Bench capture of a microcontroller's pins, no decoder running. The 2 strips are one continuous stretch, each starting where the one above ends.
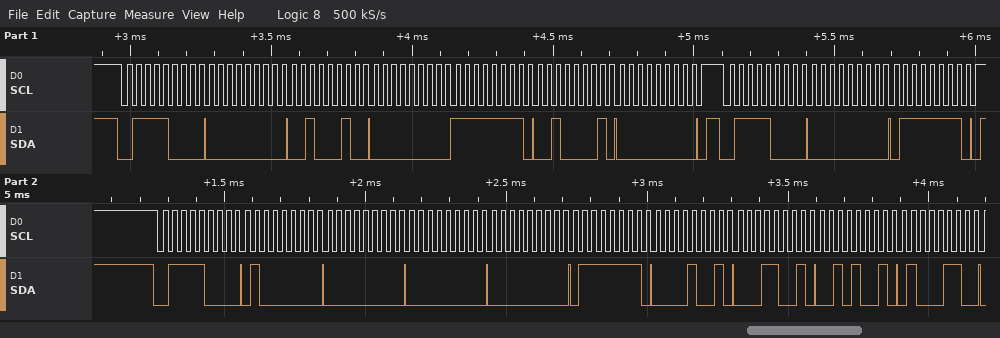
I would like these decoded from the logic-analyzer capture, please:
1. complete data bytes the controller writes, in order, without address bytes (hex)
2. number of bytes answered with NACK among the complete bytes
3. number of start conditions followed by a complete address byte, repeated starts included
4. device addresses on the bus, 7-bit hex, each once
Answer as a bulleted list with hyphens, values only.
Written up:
- 00 22 00 FF 21 00 00 7F 40 00 00 00 7F 09 19 29 46
- 0
- 3
- 0x3C
